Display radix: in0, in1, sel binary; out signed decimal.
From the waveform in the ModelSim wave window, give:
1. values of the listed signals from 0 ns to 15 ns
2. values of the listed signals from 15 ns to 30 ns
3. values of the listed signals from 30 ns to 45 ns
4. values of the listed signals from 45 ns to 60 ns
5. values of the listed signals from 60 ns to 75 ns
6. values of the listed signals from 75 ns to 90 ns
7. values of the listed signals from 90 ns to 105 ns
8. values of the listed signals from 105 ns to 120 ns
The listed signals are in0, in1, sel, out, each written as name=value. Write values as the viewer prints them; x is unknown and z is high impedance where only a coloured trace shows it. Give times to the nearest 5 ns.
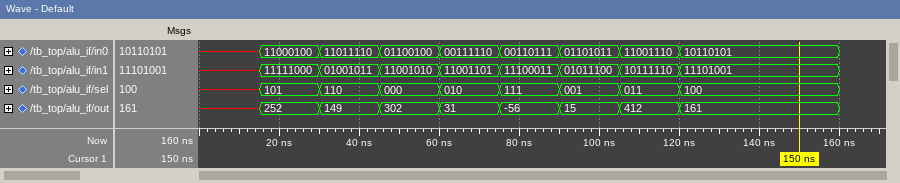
in0=x, in1=x, sel=x, out=x
in0=11000100, in1=11111000, sel=101, out=252
in0=11011110, in1=01001011, sel=110, out=149
in0=01100100, in1=11001010, sel=000, out=302
in0=00111110, in1=11001101, sel=010, out=31
in0=00110111, in1=11100011, sel=111, out=-56
in0=01101011, in1=01011100, sel=001, out=15
in0=11001110, in1=10111110, sel=011, out=412
